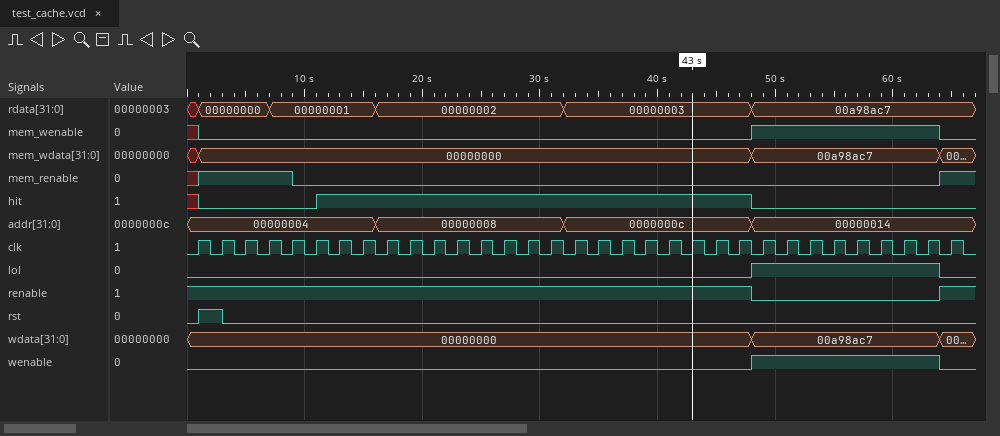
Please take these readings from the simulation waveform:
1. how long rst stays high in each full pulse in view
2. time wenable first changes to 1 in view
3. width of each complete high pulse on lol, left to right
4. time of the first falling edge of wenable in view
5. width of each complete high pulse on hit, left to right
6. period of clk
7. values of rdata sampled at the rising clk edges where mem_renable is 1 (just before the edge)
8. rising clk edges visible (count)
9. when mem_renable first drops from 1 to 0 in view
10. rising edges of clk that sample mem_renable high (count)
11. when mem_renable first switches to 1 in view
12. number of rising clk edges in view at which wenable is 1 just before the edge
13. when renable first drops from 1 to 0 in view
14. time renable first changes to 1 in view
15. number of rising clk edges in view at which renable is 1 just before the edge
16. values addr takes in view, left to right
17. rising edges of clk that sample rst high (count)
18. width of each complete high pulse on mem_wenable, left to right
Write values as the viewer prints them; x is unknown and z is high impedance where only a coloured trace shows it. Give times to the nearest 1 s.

2 s
48 s
16 s
64 s
37 s
2 s
00000000, 00000000, 00000000, 00000001, 00a98ac7
33
9 s
5
1 s
8
48 s
64 s
25
00000004, 00000008, 0000000c, 00000014
1
16 s
